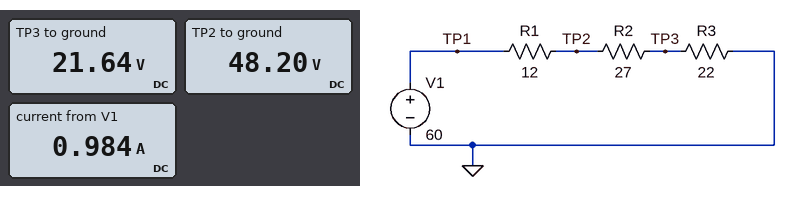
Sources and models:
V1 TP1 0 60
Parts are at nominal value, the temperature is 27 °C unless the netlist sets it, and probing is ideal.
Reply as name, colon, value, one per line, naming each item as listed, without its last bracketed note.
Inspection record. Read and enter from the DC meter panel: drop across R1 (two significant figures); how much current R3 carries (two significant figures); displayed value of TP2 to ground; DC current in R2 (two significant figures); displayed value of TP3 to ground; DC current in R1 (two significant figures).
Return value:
drop across R1: 12 V
how much current R3 carries: 980 mA
displayed value of TP2 to ground: 48.20 V
DC current in R2: 980 mA
displayed value of TP3 to ground: 21.64 V
DC current in R1: 980 mA
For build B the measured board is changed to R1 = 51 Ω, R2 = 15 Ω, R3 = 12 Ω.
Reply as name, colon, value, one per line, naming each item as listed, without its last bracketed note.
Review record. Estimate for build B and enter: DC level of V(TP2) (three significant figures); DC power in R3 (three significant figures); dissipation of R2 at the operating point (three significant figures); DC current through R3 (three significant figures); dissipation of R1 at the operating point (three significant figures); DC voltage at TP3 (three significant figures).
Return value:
DC level of V(TP2): 20.8 V
DC power in R3: 7.10 W
dissipation of R2 at the operating point: 8.88 W
DC current through R3: 769 mA
dissipation of R1 at the operating point: 30.2 W
DC voltage at TP3: 9.23 V
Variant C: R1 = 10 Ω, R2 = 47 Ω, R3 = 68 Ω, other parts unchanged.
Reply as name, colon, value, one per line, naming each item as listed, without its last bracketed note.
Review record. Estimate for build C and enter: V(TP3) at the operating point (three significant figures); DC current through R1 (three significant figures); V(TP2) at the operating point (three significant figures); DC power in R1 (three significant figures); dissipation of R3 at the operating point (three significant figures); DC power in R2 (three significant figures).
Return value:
V(TP3) at the operating point: 32.6 V
DC current through R1: 480 mA
V(TP2) at the operating point: 55.2 V
DC power in R1: 2.30 W
dissipation of R3 at the operating point: 15.7 W
DC power in R2: 10.8 W
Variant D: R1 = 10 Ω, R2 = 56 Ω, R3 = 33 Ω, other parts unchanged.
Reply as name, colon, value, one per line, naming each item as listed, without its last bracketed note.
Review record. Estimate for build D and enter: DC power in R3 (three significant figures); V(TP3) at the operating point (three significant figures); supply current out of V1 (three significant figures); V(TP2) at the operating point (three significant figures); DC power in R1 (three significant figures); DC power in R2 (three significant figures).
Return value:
DC power in R3: 12.1 W
V(TP3) at the operating point: 20.0 V
supply current out of V1: 606 mA
V(TP2) at the operating point: 53.9 V
DC power in R1: 3.67 W
DC power in R2: 20.6 W
